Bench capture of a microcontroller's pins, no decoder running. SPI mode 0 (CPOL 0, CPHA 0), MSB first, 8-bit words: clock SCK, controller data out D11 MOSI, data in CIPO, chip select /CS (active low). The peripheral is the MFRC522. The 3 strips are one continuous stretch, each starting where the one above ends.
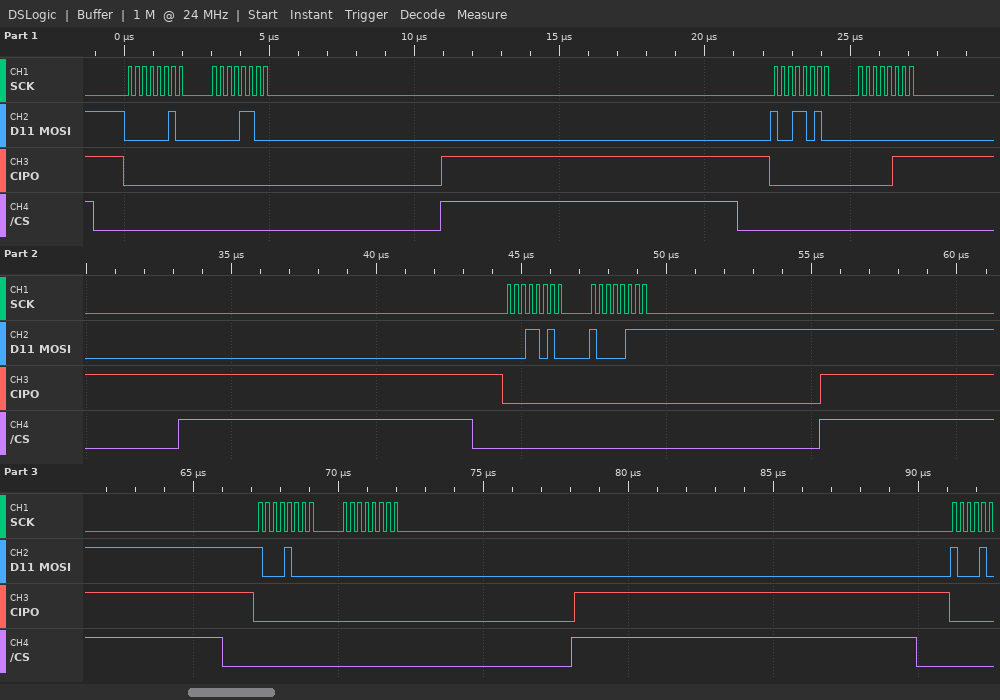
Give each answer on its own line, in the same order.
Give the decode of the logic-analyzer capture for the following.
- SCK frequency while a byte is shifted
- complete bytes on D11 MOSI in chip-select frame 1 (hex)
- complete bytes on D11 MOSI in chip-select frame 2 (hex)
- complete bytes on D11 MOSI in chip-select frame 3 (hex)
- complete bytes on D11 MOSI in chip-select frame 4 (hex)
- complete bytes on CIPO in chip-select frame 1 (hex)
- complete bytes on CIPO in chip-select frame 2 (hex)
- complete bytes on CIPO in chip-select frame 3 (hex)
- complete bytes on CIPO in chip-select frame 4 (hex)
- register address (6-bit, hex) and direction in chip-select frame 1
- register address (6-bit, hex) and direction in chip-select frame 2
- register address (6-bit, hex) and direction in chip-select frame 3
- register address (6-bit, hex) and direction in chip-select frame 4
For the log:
4 MHz
0x02 0x0C
0x9A 0x00
0x1A 0x87
0x88 0x00
0x00 0x00
0x00 0x07
0x00 0x00
0x00 0x00
0x01 write
0x0D read
0x0D write
0x04 read
